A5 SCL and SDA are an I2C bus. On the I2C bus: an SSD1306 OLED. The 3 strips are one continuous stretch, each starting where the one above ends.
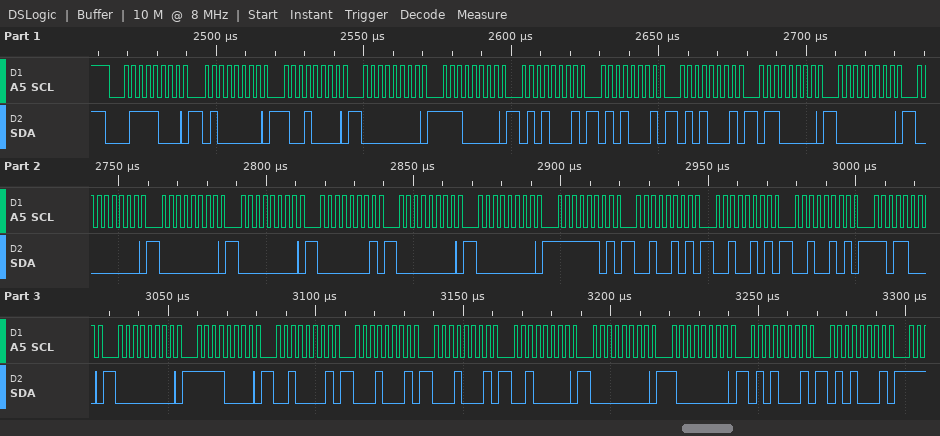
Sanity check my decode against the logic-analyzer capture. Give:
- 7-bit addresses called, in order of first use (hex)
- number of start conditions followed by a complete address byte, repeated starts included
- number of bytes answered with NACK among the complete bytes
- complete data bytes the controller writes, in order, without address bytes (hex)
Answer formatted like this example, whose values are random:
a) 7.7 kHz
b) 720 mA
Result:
a) 0x3C
b) 1
c) 0
d) 40 90 00 E0 51 51 51 60 00 00 00 00 01 00 00 FD 25 25 25 D8 00 F0 21 11 11 20 00 80 51 51
